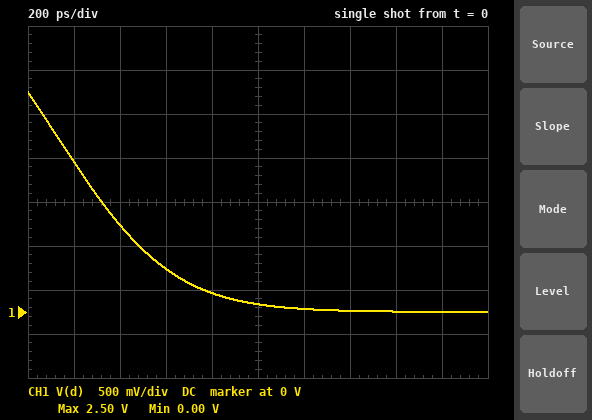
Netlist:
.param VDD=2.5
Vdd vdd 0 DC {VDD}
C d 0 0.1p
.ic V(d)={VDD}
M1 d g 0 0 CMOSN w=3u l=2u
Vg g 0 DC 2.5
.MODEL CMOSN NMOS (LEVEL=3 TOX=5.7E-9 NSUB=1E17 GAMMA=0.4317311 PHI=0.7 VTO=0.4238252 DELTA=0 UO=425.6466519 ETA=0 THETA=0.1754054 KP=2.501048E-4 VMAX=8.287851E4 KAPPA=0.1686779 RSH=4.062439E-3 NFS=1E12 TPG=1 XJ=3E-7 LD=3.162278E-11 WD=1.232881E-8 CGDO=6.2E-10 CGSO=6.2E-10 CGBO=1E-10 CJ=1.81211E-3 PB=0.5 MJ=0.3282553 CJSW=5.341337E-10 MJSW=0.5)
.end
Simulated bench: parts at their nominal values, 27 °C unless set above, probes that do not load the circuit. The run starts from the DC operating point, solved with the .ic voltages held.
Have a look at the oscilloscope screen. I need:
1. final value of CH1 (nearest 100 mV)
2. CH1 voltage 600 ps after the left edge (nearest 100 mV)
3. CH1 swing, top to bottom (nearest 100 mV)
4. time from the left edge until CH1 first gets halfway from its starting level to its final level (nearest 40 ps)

0 V
500 mV
2.5 V
320 ps
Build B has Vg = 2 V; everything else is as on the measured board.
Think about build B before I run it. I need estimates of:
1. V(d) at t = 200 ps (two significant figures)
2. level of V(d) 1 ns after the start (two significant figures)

2.0 V
310 mV
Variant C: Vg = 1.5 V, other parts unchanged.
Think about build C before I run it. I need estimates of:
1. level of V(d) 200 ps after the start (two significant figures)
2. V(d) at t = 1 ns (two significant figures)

2.2 V
1.1 V
